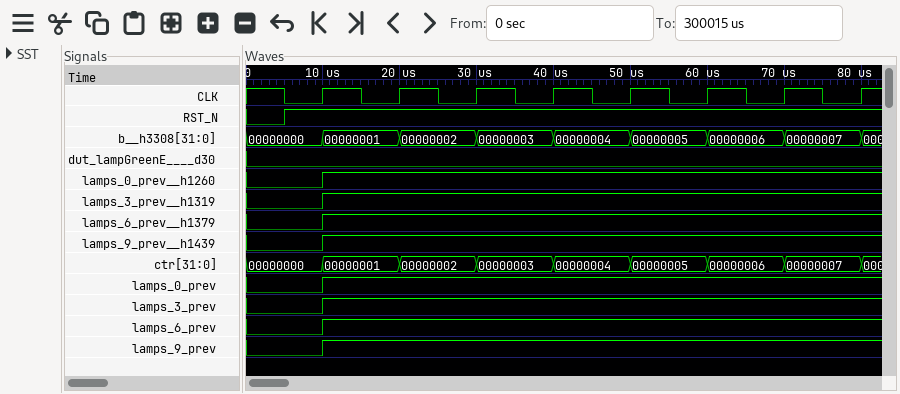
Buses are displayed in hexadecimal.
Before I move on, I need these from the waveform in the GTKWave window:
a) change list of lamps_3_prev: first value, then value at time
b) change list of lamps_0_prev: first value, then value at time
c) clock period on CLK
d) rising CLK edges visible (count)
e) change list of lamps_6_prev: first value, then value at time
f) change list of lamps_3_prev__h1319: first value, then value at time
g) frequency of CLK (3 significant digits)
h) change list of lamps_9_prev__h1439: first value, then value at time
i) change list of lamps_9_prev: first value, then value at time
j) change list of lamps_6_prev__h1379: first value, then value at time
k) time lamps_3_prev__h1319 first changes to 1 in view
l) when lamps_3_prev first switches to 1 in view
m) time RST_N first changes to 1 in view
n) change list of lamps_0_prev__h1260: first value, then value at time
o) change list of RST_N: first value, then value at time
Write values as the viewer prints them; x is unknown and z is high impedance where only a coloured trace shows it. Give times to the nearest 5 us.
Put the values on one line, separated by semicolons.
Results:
0, 1 at 10 us; 0, 1 at 10 us; 10 us; 8; 0, 1 at 10 us; 0, 1 at 10 us; 100 kHz; 0, 1 at 10 us; 0, 1 at 10 us; 0, 1 at 10 us; 10 us; 10 us; 5 us; 0, 1 at 10 us; 0, 1 at 5 us
